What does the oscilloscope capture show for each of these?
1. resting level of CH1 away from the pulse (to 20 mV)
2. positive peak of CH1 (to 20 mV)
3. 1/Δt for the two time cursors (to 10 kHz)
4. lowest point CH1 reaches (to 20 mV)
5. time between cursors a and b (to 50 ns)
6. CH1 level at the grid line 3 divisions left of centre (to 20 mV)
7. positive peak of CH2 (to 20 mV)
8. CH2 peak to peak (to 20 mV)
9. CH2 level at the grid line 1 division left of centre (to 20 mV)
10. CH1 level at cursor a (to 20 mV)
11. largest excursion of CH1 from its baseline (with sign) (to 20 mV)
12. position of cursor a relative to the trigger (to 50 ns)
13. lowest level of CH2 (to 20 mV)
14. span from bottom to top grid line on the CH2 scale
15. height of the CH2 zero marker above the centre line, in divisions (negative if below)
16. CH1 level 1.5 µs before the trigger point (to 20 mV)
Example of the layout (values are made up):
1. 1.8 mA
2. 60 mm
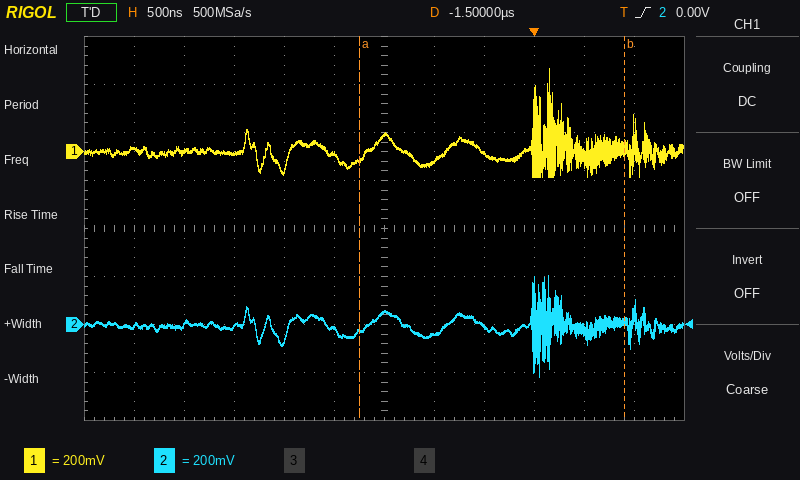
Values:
1. 0 mV
2. 340 mV
3. 380 kHz
4. -100 mV
5. 2.65 µs
6. 0 mV
7. 200 mV
8. 420 mV
9. -20 mV
10. -40 mV
11. +340 mV
12. -1.75 µs
13. -220 mV
14. 1.6 V
15. -2.0 div
16. 60 mV
